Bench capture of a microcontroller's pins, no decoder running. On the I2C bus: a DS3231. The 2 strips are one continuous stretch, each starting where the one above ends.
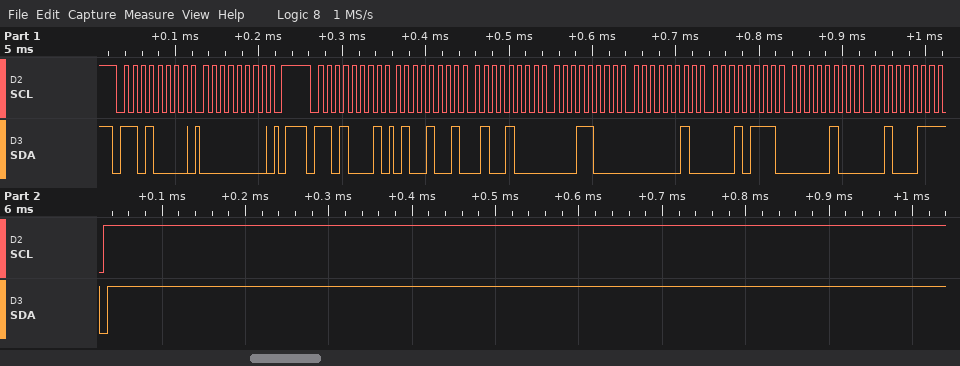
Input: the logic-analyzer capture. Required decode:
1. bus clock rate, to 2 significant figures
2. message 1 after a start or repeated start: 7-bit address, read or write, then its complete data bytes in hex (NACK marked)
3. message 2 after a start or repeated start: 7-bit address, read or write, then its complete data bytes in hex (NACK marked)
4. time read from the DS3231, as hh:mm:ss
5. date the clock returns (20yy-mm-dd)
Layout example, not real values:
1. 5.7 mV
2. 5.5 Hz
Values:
1. 100 kHz
2. 0x68 write: 00
3. 0x68 read: 49 48 18 02 17 04 23 NACK
4. 18:48:49
5. 2023-04-17
